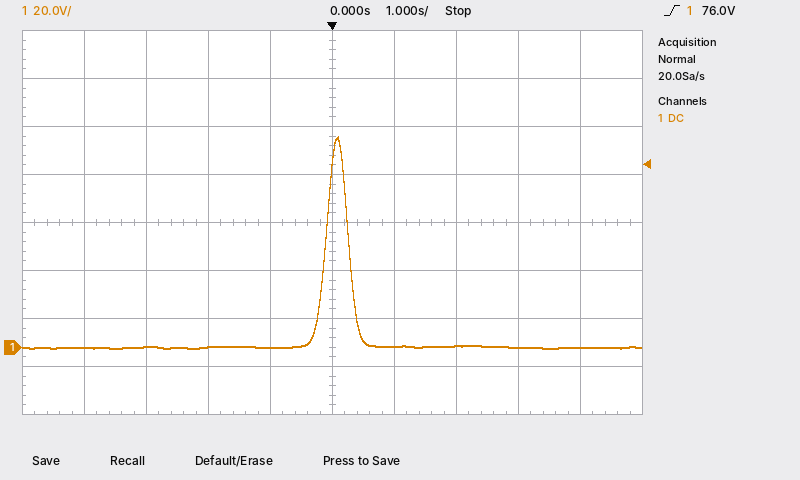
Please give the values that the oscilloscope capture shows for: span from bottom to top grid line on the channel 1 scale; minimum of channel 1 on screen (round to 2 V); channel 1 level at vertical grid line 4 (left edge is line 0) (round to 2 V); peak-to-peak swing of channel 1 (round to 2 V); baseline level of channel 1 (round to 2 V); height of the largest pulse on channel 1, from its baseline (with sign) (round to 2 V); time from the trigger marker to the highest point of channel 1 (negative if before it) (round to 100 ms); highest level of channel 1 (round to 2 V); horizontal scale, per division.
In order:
160 V
0 V
0 V
88 V
0 V
+88 V
+100 ms
88 V
1 s
